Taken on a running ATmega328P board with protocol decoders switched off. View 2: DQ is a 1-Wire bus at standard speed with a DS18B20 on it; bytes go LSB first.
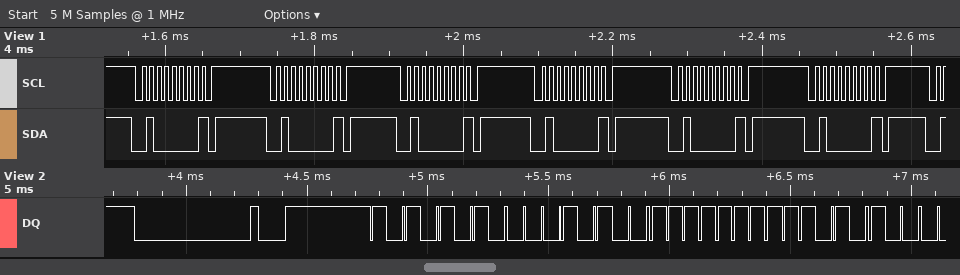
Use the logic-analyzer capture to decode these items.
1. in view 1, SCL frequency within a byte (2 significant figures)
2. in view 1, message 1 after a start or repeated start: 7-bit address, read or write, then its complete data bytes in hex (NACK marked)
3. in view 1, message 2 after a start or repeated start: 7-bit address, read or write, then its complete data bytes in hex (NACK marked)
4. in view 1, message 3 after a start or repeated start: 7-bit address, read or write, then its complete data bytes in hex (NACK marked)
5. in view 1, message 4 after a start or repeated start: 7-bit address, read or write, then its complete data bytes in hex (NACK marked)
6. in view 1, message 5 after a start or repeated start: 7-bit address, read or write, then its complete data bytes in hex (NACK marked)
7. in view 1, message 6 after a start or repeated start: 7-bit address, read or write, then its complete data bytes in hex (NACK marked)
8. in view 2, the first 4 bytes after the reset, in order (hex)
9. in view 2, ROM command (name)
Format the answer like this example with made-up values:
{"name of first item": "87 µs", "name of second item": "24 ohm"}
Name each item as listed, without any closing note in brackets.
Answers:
{"in view 1, SCL frequency within a byte": "100 kHz", "in view 1, message 1 after a start or repeated start: 7-bit address, read or write, then its complete data bytes in hex": "0x20 write NACK", "in view 1, message 2 after a start or repeated start: 7-bit address, read or write, then its complete data bytes in hex": "0x20 write NACK", "in view 1, message 3 after a start or repeated start: 7-bit address, read or write, then its complete data bytes in hex": "0x20 write NACK", "in view 1, message 4 after a start or repeated start: 7-bit address, read or write, then its complete data bytes in hex": "0x20 write NACK", "in view 1, message 5 after a start or repeated start: 7-bit address, read or write, then its complete data bytes in hex": "0x20 write NACK", "in view 1, message 6 after a start or repeated start: 7-bit address, read or write, then its complete data bytes in hex": "0x20 write NACK", "in view 2, the first 4 bytes after the reset, in order": "55 28 FF 2B", "in view 2, ROM command": "Match ROM"}
